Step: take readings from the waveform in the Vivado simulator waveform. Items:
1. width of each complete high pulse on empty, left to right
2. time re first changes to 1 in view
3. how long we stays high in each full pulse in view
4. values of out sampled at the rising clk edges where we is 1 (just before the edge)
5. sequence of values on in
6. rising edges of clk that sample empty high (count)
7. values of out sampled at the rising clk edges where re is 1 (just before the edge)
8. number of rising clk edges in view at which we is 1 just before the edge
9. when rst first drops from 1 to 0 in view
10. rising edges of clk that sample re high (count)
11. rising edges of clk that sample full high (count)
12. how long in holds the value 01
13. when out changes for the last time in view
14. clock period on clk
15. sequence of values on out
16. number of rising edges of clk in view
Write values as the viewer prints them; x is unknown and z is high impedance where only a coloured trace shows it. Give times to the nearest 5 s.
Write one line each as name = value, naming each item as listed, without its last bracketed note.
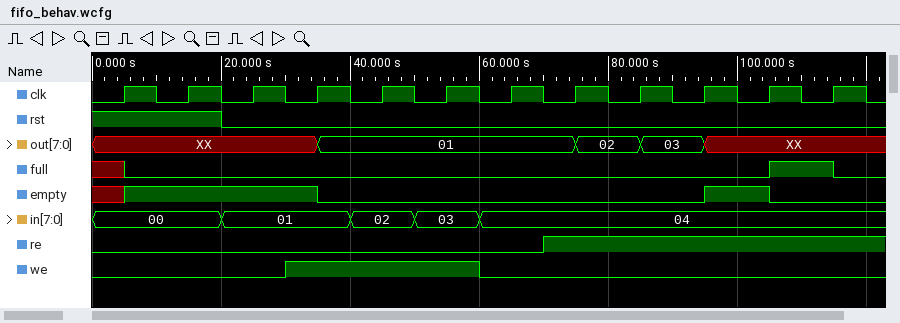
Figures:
width of each complete high pulse on empty, left to right = 10 s
time re first changes to 1 in view = 70 s
how long we stays high in each full pulse in view = 30 s
values of out sampled at the rising clk edges where we is 1 = XX, 01, 01
sequence of values on in = 00, 01, 02, 03, 04
rising edges of clk that sample empty high = 4
values of out sampled at the rising clk edges where re is 1 = 01, 02, 03, XX, XX
number of rising clk edges in view at which we is 1 just before the edge = 3
when rst first drops from 1 to 0 in view = 20 s
rising edges of clk that sample re high = 5
rising edges of clk that sample full high = 1
how long in holds the value 01 = 20 s
when out changes for the last time in view = 95 s
clock period on clk = 10 s
sequence of values on out = XX, 01, 02, 03, XX
number of rising edges of clk in view = 12
